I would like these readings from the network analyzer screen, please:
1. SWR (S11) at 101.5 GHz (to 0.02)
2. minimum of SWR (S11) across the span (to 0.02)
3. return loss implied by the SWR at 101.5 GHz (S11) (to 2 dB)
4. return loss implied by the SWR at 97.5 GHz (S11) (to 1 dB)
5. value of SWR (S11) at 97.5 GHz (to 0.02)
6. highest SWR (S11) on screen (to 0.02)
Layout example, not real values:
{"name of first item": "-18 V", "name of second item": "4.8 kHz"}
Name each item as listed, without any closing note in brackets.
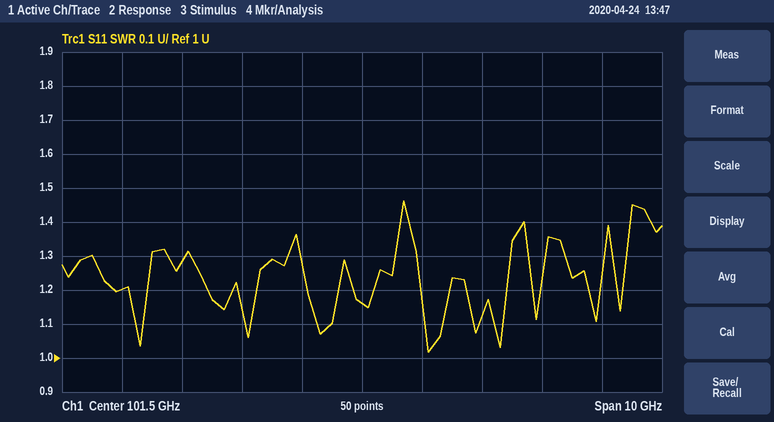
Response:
{"SWR (S11) at 101.5 GHz": "1.16", "minimum of SWR (S11) across the span": "1.02", "return loss implied by the SWR at 101.5 GHz (S11)": "22 dB", "return loss implied by the SWR at 97.5 GHz (S11)": "21 dB", "value of SWR (S11) at 97.5 GHz": "1.20", "highest SWR (S11) on screen": "1.46"}
